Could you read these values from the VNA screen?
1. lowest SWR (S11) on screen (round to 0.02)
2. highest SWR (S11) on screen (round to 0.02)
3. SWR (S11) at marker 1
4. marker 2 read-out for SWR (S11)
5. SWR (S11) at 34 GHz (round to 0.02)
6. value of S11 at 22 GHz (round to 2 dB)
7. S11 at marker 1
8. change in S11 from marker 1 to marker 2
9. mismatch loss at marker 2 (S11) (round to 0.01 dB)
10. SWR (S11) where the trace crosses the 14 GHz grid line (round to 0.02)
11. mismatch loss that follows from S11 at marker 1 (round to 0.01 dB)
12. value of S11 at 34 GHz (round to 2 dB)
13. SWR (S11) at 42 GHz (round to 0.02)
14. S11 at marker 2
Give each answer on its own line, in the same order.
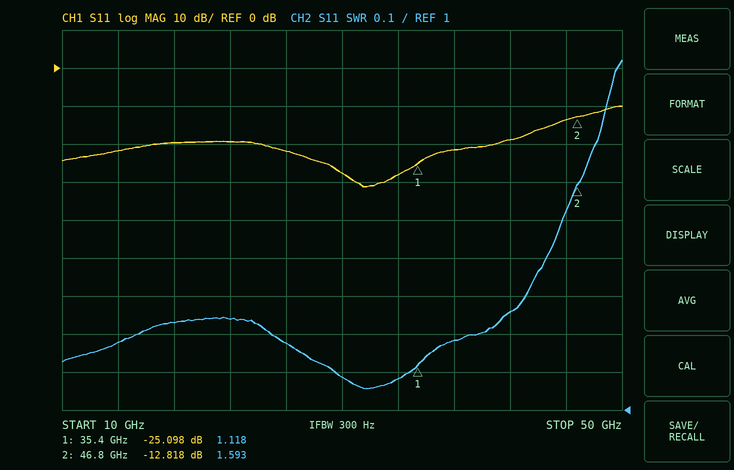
1.06
1.92
1.118
1.593
1.08
-20 dB
-25.098 dB
12.280 dB
0.23 dB
1.18
0.01 dB
-28 dB
1.26
-12.818 dB
